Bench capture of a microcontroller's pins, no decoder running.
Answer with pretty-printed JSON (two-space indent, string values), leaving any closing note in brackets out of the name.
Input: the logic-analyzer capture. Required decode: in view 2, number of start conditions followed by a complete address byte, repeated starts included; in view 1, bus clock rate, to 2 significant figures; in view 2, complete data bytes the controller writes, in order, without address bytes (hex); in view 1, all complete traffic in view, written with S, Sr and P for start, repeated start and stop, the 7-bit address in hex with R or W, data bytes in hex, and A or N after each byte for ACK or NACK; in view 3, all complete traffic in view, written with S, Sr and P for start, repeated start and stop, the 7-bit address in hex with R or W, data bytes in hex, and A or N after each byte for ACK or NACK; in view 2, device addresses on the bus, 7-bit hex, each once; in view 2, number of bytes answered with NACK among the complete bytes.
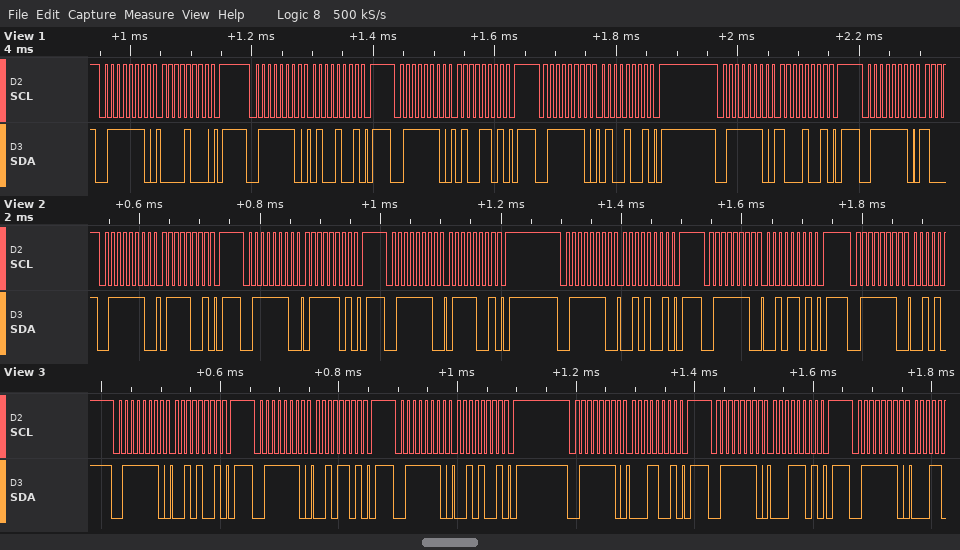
{
  "in view 2, number of start conditions followed by a complete address byte, repeated starts included": "6",
  "in view 1, bus clock rate, to 2 significant figures": "100 kHz",
  "in view 2, complete data bytes the controller writes, in order, without address bytes": "79 7D 79 29 2D",
  "in view 1, all complete traffic in view, written with S, Sr and P for start, repeated start and stop, the 7-bit address in hex with R or W, data bytes in hex, and A or N after each byte for ACK or NACK": "S 3FW A 08 A P S 3FW A 49 A P S 3FW A 4D A P S 3FW A 49 A P S 3FW A 89 A P S 3FW A",
  "in view 3, all complete traffic in view, written with S, Sr and P for start, repeated start and stop, the 7-bit address in hex with R or W, data bytes in hex, and A or N after each byte for ACK or NACK": "S 3FW A 29 A P S 3FW A 2D A P S 3FW A 29 A P S 3FW A 19 A P S 3FW A 1D A P S 3FW A",
  "in view 2, device addresses on the bus, 7-bit hex, each once": "0x3F",
  "in view 2, number of bytes answered with NACK among the complete bytes": "0"
}
